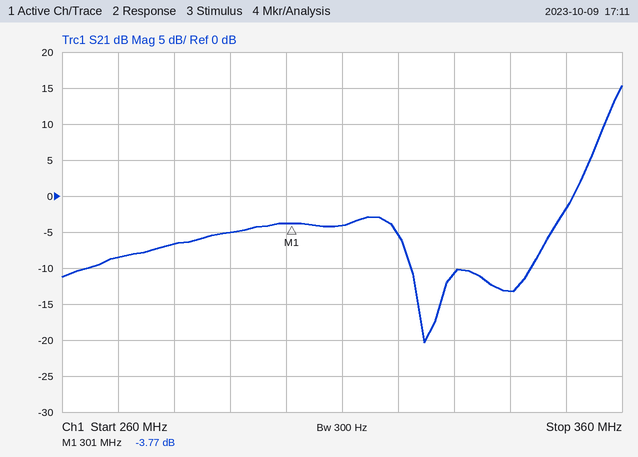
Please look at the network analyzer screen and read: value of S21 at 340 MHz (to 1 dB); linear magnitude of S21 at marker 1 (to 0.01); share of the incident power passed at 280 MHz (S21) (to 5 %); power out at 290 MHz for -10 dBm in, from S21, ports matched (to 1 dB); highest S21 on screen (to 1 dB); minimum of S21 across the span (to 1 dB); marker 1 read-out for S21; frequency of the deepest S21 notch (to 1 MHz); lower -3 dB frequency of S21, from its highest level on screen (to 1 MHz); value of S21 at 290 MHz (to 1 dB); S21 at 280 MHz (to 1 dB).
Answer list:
-13 dB
0.65
20 %
-15 dBm
15 dB
-20 dB
-3.77 dB
325 MHz
358 MHz
-5 dB
-7 dB
